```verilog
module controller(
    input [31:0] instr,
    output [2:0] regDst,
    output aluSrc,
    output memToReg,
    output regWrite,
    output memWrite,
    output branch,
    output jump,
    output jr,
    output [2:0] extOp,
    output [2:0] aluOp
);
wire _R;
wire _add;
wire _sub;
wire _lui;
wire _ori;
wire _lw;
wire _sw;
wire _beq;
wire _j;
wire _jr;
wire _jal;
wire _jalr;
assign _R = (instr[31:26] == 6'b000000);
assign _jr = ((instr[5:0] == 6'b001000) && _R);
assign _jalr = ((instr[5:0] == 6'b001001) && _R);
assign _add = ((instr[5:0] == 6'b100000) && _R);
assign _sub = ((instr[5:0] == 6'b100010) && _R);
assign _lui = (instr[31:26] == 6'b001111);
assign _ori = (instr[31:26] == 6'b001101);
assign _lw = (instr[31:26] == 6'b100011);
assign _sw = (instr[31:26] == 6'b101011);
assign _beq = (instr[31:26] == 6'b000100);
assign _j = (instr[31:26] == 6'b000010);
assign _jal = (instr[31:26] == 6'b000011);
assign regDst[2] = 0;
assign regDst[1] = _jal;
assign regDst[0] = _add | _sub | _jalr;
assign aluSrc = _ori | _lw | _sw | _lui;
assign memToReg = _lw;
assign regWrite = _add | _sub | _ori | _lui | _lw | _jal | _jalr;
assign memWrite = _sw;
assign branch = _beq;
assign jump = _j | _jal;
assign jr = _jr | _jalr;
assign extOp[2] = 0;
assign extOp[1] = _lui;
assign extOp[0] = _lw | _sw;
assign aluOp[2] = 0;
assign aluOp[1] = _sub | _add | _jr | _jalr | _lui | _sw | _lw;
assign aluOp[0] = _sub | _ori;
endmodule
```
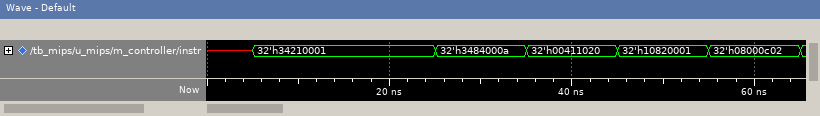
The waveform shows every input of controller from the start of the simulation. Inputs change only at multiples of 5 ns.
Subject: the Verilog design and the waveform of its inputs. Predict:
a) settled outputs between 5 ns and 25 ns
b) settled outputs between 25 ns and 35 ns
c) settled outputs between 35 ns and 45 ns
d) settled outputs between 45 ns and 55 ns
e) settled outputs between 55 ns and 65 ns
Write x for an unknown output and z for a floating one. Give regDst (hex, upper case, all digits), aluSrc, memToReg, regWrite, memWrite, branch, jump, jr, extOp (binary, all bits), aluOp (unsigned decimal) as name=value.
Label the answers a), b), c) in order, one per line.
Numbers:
a) regDst=0, aluSrc=1, memToReg=0, regWrite=1, memWrite=0, branch=0, jump=0, jr=0, extOp=000, aluOp=1
b) regDst=0, aluSrc=1, memToReg=0, regWrite=1, memWrite=0, branch=0, jump=0, jr=0, extOp=000, aluOp=1
c) regDst=1, aluSrc=0, memToReg=0, regWrite=1, memWrite=0, branch=0, jump=0, jr=0, extOp=000, aluOp=2
d) regDst=0, aluSrc=0, memToReg=0, regWrite=0, memWrite=0, branch=1, jump=0, jr=0, extOp=000, aluOp=0
e) regDst=0, aluSrc=0, memToReg=0, regWrite=0, memWrite=0, branch=0, jump=1, jr=0, extOp=000, aluOp=0
